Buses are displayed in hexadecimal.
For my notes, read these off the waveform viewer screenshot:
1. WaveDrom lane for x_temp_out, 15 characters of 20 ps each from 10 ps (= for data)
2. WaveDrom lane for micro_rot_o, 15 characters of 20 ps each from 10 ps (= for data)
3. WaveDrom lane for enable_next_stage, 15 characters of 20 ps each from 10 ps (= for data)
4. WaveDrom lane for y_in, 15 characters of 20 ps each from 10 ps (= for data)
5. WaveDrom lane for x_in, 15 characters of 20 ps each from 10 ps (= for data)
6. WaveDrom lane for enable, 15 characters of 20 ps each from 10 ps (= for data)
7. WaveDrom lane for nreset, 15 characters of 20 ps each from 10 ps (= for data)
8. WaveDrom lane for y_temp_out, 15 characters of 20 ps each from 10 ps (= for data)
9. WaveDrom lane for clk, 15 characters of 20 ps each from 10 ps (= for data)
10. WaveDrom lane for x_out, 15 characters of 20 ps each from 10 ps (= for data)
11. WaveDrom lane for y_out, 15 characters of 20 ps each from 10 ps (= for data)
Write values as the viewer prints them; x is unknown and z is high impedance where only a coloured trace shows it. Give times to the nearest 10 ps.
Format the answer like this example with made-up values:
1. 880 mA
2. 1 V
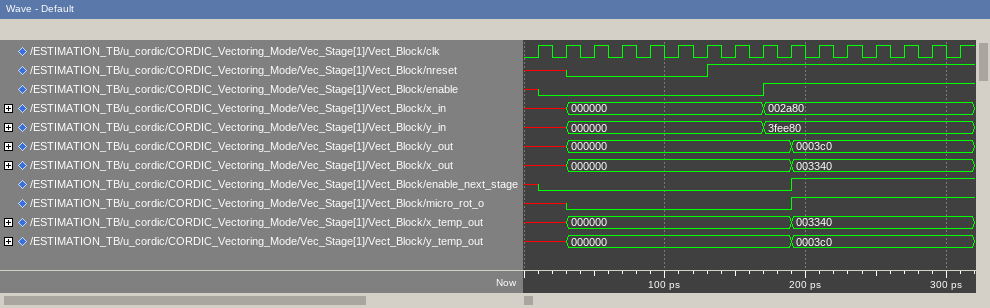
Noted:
1. {name: 'x_temp_out', wave: 'x=.......=.....', data: '000000 003340'}
2. {name: 'micro_rot_o', wave: 'x0.......1.....'}
3. {name: 'enable_next_stage', wave: '0........1.....'}
4. {name: 'y_in', wave: 'x=......=......', data: '000000 3fee80'}
5. {name: 'x_in', wave: 'x=......=......', data: '000000 002a80'}
6. {name: 'enable', wave: '0.......1......'}
7. {name: 'nreset', wave: 'x0....1........'}
8. {name: 'y_temp_out', wave: 'x=.......=.....', data: '000000 0003c0'}
9. {name: 'clk', wave: 'p..............'}
10. {name: 'x_out', wave: 'x=.......=.....', data: '000000 003340'}
11. {name: 'y_out', wave: 'x=.......=.....', data: '000000 0003c0'}
